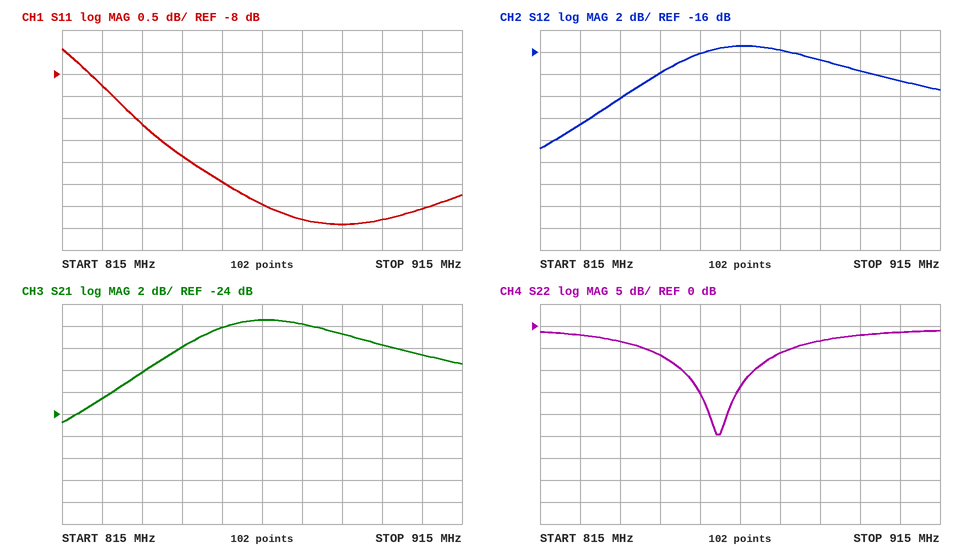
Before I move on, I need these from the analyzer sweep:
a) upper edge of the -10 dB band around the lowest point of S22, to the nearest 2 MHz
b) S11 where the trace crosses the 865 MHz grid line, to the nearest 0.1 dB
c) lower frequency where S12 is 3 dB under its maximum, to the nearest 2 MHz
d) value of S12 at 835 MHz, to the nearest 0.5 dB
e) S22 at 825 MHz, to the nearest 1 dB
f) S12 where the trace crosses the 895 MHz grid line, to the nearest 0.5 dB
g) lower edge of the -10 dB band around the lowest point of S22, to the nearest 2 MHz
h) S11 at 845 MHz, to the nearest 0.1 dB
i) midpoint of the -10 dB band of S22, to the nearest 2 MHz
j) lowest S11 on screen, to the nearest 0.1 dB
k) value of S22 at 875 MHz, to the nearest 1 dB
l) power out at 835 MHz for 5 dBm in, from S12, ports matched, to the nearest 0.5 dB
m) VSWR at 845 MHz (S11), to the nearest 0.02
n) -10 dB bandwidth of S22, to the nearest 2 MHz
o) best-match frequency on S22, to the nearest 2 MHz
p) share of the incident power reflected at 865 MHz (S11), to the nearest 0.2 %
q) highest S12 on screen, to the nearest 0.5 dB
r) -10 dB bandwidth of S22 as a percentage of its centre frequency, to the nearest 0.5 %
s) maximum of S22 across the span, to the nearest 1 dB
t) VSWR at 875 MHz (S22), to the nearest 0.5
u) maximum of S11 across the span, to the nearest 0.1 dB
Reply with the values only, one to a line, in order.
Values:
868 MHz
-11.0 dB
842 MHz
-20.0 dB
-2 dB
-17.5 dB
850 MHz
-9.9 dB
860 MHz
-11.4 dB
-6 dB
-15.0 dBm
1.94
18 MHz
860 MHz
8.0 %
-15.5 dB
2.0 %
-1 dB
3.0
-7.4 dB
